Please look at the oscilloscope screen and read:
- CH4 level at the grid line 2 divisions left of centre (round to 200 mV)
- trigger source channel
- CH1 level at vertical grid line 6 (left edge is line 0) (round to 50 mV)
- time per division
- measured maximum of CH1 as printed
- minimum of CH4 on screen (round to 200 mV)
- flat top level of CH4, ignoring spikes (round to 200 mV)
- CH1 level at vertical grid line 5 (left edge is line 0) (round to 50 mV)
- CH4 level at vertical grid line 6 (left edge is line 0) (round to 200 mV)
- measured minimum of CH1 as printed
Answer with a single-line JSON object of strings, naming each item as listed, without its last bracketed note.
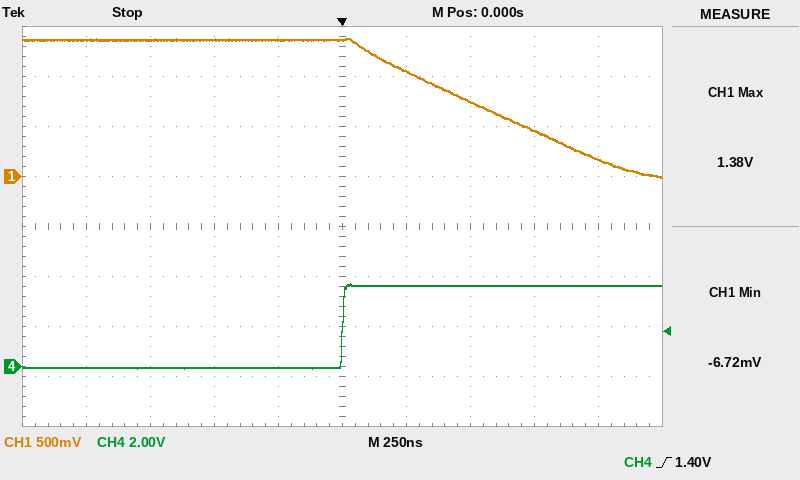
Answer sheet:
{"CH4 level at the grid line 2 divisions left of centre": "0.0 V", "trigger source channel": "CH4", "CH1 level at vertical grid line 6 (left edge is line 0)": "1.05 V", "time per division": "250 ns", "measured maximum of CH1 as printed": "1.38 V", "minimum of CH4 on screen": "0.0 V", "flat top level of CH4, ignoring spikes": "3.2 V", "CH1 level at vertical grid line 5 (left edge is line 0)": "1.35 V", "CH4 level at vertical grid line 6 (left edge is line 0)": "3.2 V", "measured minimum of CH1 as printed": "-6.72 mV"}
